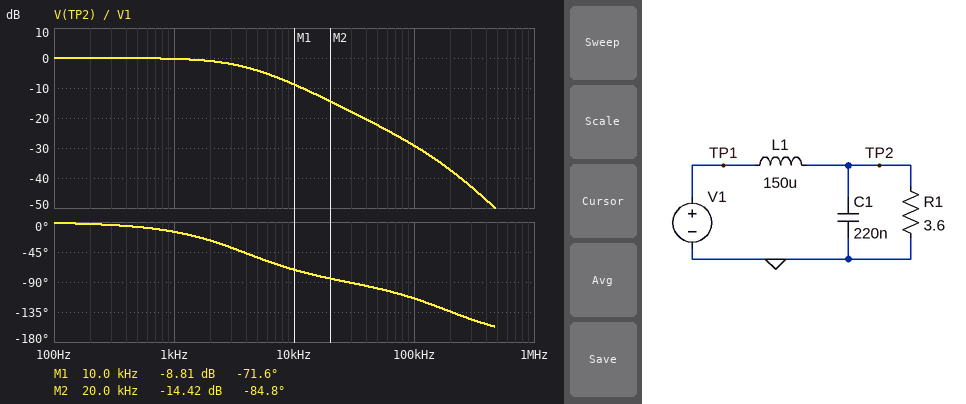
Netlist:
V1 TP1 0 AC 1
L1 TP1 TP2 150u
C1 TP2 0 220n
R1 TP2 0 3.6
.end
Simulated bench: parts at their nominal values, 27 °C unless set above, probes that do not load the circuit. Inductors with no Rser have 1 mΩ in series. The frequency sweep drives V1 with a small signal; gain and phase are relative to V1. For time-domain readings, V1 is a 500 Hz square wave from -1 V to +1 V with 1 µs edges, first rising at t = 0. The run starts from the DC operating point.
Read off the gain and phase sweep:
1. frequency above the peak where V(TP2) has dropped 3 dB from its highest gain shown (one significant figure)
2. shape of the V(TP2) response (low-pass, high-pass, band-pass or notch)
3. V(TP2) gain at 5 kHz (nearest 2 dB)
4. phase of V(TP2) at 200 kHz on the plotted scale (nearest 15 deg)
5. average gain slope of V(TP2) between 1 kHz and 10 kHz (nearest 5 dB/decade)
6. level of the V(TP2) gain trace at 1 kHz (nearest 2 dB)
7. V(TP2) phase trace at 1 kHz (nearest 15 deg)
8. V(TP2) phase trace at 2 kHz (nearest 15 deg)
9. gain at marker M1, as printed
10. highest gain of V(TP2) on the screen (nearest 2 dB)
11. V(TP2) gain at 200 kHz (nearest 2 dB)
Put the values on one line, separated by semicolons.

4 kHz; low-pass; -4 dB; -135 deg; -10 dB/decade; 0 dB; -15 deg; -30 deg; -8.81 dB; 0 dB; -38 dB
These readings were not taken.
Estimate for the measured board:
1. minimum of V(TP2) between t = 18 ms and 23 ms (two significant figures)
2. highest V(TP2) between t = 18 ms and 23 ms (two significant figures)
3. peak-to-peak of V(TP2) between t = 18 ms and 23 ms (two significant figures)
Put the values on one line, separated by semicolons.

-1.0 V; 1.0 V; 2.0 V
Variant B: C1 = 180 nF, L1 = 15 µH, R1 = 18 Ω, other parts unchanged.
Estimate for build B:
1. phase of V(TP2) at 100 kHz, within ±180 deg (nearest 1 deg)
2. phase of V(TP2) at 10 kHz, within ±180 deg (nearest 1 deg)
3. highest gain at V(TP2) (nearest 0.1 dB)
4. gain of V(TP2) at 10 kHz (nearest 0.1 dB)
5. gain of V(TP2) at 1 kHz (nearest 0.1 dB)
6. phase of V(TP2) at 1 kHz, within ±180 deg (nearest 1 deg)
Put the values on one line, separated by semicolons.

-97 deg; -3 deg; 6.2 dB; 0.1 dB; 0 dB; 0 deg
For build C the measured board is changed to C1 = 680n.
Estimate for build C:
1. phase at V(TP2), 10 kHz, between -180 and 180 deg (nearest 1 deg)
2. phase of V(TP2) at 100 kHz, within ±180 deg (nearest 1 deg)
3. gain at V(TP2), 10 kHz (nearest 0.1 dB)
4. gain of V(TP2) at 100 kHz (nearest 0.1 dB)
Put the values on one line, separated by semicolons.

-77 deg; -146 deg; -8.6 dB; -33.5 dB
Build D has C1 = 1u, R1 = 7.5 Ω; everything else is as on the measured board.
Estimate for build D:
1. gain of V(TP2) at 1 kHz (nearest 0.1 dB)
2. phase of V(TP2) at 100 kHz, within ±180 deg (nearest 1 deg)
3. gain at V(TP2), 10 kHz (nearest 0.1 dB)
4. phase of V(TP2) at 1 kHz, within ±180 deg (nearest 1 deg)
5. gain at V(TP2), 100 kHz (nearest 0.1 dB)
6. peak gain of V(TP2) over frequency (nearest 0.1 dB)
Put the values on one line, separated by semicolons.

0 dB; -168 deg; -2.4 dB; -7 deg; -35.5 dB; 0 dB
